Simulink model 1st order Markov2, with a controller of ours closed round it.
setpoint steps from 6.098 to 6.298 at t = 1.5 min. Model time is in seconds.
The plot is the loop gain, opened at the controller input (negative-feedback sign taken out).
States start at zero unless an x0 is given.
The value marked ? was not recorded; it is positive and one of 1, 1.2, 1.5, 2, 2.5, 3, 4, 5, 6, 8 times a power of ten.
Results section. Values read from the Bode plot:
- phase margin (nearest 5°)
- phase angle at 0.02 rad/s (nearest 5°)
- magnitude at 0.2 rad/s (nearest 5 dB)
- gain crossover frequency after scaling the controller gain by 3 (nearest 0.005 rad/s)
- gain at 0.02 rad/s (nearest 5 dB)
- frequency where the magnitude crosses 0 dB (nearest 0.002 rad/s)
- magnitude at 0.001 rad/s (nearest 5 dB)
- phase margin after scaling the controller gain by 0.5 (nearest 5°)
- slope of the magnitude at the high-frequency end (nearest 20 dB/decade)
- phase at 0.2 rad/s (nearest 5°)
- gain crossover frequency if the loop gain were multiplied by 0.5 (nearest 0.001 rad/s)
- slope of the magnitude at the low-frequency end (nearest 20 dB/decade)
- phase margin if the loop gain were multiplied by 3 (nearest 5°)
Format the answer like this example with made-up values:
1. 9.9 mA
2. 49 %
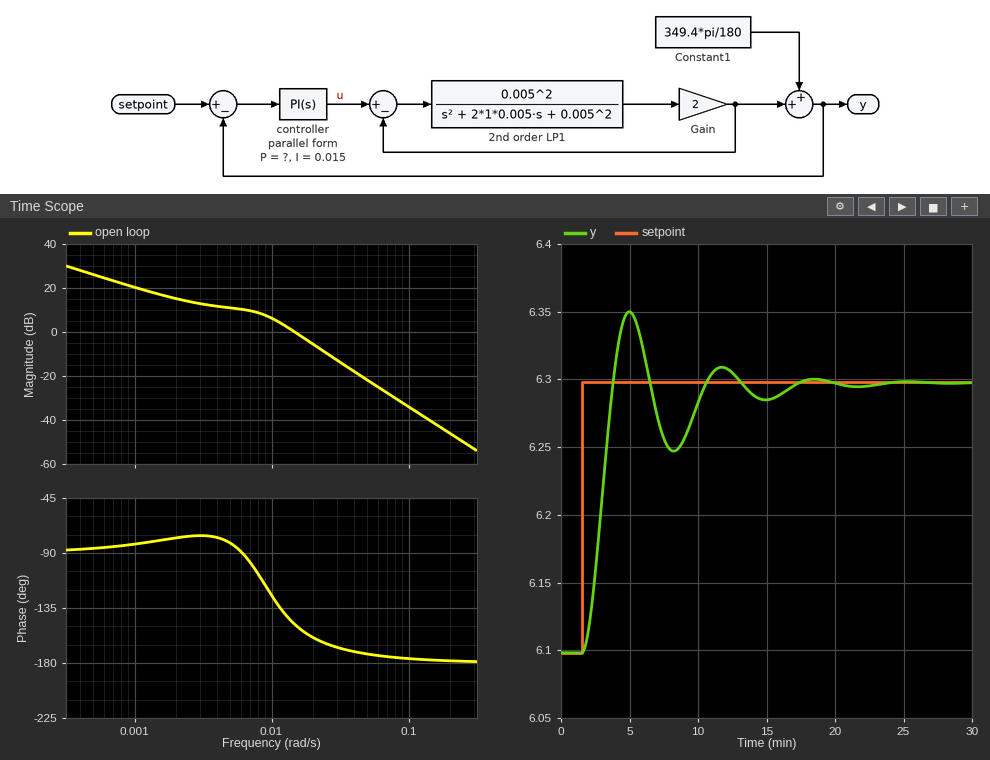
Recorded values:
1. 30°
2. -160°
3. -45 dB
4. 0.025 rad/s
5. -5 dB
6. 0.014 rad/s
7. 20 dB
8. 55°
9. -40 dB/decade
10. -180°
11. 0.010 rad/s
12. -20 dB/decade
13. 15°
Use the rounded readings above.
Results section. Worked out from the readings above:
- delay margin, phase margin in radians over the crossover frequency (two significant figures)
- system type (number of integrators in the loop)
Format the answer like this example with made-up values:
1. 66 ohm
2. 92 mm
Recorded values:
1. 37 s
2. 1
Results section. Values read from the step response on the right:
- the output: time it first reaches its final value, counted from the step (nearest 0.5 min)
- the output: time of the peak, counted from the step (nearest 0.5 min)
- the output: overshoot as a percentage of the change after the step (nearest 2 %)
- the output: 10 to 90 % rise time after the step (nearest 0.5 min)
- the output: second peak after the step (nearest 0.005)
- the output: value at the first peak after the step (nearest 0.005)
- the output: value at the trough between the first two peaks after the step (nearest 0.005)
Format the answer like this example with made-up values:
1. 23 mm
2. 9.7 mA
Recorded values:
1. 2.5 min
2. 3.5 min
3. 26 %
4. 1.5 min
5. 6.310
6. 6.350
7. 6.245
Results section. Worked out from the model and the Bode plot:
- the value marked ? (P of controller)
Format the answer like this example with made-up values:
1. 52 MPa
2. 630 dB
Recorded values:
1. 4
